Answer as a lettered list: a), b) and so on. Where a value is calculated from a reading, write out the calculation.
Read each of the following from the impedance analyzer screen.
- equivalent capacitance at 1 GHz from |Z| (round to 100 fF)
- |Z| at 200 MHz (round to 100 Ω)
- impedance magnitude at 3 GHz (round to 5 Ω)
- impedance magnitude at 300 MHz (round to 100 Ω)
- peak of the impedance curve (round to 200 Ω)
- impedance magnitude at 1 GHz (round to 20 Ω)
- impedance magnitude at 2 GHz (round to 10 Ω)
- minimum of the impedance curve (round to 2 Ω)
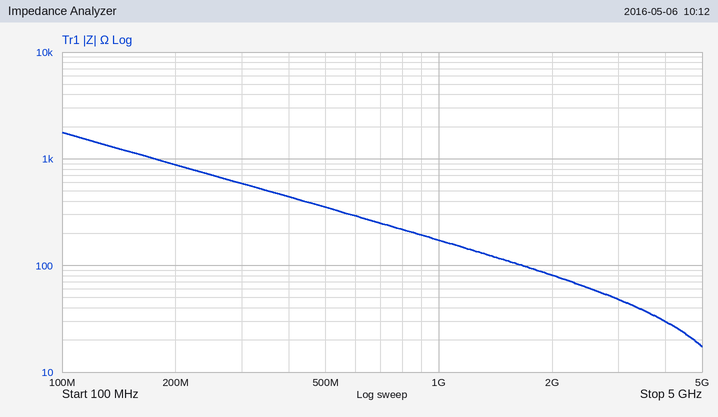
a) C = 1/(2π × 1 GHz × 180 Ω) ≈ 884 fF, so 900 fF to the nearest 100 fF
b) 900 Ω
c) 50 Ω
d) 600 Ω
e) 1.8 kΩ
f) 180 Ω
g) 80 Ω
h) 18 Ω
